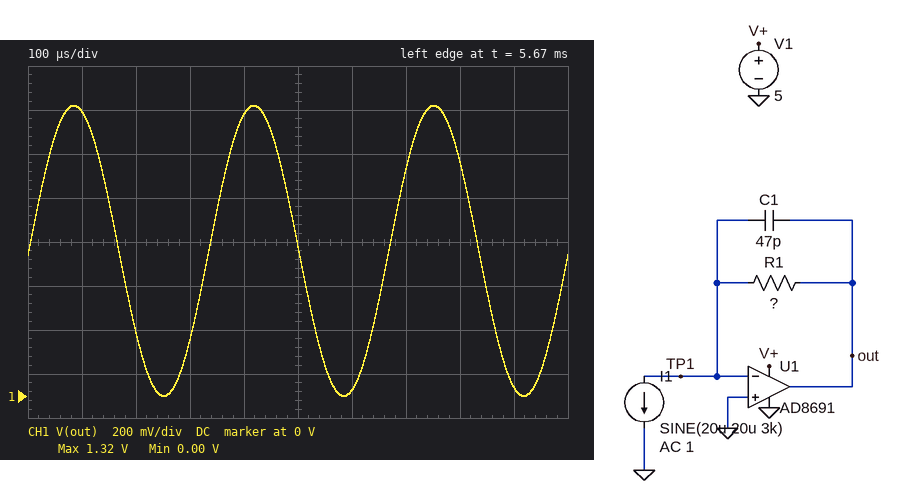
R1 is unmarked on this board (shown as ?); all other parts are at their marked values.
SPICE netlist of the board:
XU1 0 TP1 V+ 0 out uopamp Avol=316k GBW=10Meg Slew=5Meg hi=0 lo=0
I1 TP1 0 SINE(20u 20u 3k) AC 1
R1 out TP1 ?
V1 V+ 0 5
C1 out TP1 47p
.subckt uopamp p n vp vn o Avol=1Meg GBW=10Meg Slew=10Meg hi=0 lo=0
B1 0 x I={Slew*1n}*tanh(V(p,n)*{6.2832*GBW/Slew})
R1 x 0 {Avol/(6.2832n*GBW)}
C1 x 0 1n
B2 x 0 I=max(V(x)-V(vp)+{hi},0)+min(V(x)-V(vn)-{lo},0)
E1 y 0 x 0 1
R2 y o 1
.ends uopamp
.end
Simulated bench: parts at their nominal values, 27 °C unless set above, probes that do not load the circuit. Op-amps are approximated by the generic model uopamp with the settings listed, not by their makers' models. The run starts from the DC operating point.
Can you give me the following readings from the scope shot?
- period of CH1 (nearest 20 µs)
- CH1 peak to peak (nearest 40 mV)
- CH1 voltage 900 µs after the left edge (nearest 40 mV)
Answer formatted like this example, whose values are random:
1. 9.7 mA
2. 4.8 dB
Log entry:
1. 340 µs
2. 1.32 V
3. 40 mV
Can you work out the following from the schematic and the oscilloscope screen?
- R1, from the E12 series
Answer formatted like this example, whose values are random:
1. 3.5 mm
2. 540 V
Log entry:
1. 33 kΩ
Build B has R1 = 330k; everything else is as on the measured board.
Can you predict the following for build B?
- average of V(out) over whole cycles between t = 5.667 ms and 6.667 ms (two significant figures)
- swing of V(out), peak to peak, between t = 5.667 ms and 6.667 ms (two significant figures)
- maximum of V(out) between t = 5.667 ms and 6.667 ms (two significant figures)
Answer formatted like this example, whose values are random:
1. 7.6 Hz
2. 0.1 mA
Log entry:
1. 3.7 V
2. 4.7 V
3. 5.0 V
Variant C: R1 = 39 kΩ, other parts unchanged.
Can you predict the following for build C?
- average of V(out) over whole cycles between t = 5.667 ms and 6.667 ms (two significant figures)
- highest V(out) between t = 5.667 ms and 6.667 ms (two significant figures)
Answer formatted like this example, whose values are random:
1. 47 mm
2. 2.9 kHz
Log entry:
1. 780 mV
2. 1.6 V
